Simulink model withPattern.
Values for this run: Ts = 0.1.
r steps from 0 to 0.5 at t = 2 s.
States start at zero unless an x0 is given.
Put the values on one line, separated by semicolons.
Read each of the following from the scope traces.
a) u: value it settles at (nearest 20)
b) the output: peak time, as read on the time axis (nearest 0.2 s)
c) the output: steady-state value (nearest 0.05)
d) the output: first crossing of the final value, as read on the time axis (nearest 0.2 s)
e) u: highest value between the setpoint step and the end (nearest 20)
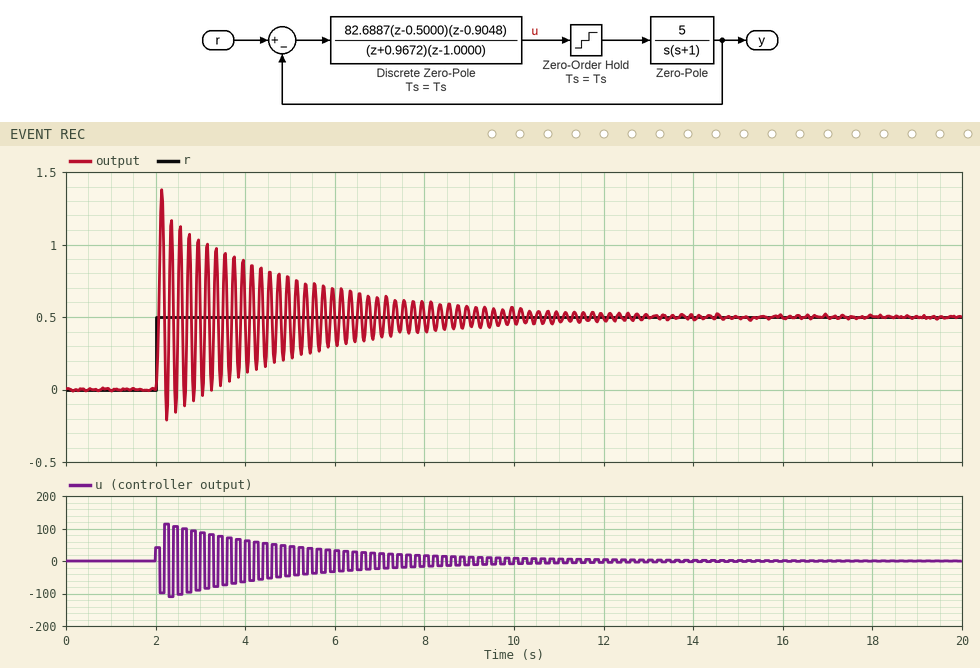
0; 2.2 s; 0.50; 2.0 s; 120
